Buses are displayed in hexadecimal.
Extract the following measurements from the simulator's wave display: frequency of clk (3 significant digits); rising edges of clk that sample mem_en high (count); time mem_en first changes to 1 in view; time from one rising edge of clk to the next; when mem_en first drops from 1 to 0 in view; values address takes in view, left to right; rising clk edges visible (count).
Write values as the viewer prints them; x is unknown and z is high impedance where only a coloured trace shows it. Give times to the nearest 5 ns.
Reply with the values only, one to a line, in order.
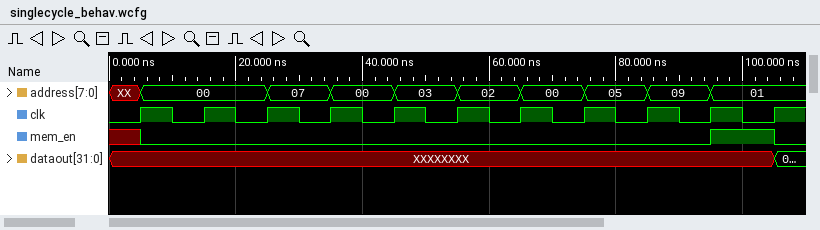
100 MHz
1
95 ns
10 ns
105 ns
XX, 00, 07, 00, 03, 02, 00, 05, 09, 01
11
